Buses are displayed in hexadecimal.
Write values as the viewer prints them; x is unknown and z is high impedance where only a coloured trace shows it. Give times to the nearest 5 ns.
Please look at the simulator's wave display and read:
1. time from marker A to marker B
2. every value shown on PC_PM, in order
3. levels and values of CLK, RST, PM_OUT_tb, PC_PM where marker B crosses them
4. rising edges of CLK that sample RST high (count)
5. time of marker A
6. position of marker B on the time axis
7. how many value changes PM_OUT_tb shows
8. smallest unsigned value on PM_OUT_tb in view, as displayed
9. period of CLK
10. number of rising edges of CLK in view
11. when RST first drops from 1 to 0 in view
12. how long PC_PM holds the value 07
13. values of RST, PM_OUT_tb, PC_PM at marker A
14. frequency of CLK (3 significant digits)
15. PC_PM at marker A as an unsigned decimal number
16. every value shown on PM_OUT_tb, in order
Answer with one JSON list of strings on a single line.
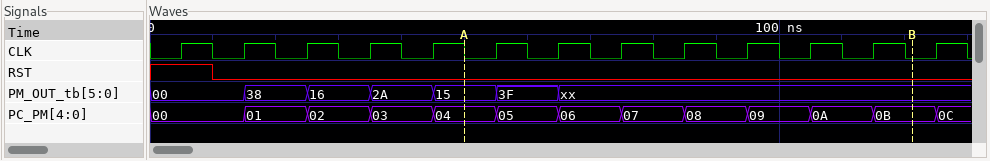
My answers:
["70 ns", "00, 01, 02, 03, 04, 05, 06, 07, 08, 09, 0A, 0B, 0C", "CLK=0, RST=0, PM_OUT_tb=xx, PC_PM=0B", "1", "50 ns", "120 ns", "6", "00", "10 ns", "13", "10 ns", "10 ns", "RST=0, PM_OUT_tb=15, PC_PM=04", "100 MHz", "4", "00, 38, 16, 2A, 15, 3F, xx"]
